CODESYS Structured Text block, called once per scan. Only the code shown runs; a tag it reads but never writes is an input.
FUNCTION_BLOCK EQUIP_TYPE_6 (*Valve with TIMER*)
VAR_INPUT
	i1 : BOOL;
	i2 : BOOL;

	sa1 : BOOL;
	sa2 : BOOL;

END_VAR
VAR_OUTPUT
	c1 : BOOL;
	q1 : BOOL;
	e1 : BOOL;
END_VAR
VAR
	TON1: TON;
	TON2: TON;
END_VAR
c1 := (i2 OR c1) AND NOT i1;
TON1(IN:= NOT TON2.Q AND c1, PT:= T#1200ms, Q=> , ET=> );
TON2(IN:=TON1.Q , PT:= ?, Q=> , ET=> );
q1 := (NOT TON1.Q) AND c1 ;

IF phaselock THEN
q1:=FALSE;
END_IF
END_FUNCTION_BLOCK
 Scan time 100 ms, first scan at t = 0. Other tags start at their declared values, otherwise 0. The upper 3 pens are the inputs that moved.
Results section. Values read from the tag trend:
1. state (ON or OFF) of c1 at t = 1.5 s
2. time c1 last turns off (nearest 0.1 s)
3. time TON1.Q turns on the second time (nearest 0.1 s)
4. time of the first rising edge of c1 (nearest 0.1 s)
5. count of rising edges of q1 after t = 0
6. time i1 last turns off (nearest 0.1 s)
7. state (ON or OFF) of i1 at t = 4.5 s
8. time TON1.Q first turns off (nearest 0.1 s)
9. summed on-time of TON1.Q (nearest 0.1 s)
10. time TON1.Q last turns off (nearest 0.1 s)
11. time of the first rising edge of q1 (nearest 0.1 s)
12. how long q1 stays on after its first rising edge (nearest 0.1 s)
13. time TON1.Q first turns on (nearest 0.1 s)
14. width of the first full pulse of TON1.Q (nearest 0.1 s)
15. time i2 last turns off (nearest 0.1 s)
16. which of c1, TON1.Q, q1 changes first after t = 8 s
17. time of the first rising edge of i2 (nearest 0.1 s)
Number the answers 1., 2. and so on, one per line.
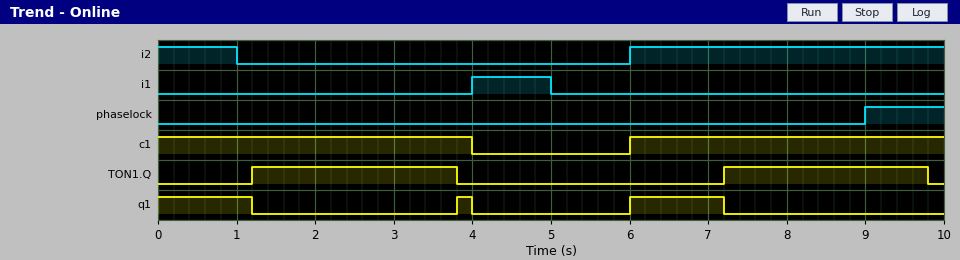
1. ON
2. 4.0 s
3. 7.2 s
4. 6.0 s
5. 2
6. 5.0 s
7. ON
8. 3.8 s
9. 5.2 s
10. 9.8 s
11. 3.8 s
12. 0.2 s
13. 1.2 s
14. 2.6 s
15. 1.0 s
16. TON1.Q
17. 6.0 s
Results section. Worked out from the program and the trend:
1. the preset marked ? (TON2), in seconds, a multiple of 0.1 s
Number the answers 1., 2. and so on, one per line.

1. 2.5 s
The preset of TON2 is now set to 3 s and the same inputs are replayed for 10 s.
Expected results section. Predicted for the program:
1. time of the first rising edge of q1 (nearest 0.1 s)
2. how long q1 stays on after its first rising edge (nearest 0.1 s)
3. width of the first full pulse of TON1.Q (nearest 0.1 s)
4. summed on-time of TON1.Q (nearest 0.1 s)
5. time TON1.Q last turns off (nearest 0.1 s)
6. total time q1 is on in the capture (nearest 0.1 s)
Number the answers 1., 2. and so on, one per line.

1. 6.0 s
2. 1.2 s
3. 2.8 s
4. 5.6 s
5. 4.0 s
6. 2.4 s
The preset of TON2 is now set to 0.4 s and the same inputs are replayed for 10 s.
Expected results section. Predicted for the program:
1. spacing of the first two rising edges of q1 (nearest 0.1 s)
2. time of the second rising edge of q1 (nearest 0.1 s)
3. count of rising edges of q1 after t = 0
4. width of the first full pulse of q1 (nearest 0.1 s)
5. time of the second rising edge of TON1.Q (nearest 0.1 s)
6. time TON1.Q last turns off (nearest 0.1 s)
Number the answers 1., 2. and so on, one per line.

1. 1.8 s
2. 3.5 s
3. 4
4. 1.3 s
5. 3.0 s
6. 9.5 s
